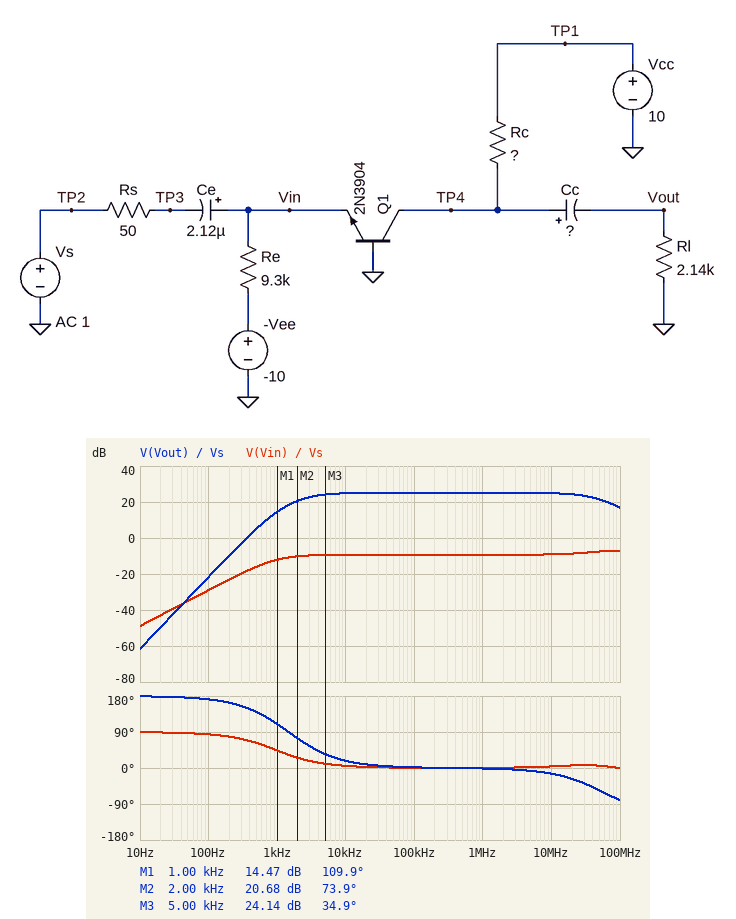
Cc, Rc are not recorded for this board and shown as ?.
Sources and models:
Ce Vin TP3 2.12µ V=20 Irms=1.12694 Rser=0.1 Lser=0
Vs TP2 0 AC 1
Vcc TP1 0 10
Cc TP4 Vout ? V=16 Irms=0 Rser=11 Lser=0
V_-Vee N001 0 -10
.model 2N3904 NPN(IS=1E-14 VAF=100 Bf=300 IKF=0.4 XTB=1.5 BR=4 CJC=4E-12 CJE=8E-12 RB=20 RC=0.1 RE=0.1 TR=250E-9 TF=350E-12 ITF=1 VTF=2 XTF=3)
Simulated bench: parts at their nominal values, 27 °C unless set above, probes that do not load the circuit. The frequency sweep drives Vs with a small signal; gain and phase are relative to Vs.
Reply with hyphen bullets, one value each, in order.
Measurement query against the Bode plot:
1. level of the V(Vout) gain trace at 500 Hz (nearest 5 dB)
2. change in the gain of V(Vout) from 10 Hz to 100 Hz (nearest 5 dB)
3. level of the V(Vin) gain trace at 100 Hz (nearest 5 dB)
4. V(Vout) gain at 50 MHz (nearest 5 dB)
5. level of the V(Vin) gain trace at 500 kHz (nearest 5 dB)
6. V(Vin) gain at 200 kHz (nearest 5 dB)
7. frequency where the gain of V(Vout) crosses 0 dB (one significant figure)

- 5 dB
- 40 dB
- -30 dB
- 20 dB
- -10 dB
- -10 dB
- 400 Hz
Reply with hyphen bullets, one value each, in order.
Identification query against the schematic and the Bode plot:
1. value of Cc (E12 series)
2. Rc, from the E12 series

- 12 nF
- 3.9 kΩ
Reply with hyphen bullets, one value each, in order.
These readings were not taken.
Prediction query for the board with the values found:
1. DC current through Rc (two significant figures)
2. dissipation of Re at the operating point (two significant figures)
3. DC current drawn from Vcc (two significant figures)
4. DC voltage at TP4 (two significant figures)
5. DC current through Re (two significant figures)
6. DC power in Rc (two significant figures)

- 1.0 mA
- 9.4 mW
- 1.0 mA
- 6.1 V
- 1.0 mA
- 3.9 mW
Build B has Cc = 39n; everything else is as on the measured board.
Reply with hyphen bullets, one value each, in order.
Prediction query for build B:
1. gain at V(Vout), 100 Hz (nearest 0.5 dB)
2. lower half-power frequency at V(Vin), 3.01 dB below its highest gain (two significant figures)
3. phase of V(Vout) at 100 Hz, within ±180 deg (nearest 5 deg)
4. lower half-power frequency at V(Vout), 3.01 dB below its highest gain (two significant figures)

- -11.5 dB
- 2.3 kHz
- 165 deg
- 1.3 kHz
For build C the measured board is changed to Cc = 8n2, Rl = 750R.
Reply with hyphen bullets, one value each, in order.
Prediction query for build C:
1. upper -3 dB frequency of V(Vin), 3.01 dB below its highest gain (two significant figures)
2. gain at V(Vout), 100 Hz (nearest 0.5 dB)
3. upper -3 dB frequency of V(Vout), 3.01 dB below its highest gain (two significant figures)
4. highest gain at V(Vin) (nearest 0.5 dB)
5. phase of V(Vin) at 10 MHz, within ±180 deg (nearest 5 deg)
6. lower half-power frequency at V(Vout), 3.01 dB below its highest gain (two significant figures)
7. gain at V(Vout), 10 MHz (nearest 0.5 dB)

- 1.3 GHz
- -34.0 dB
- 84 MHz
- -7.5 dB
- 0 deg
- 4.4 kHz
- 18.0 dB
